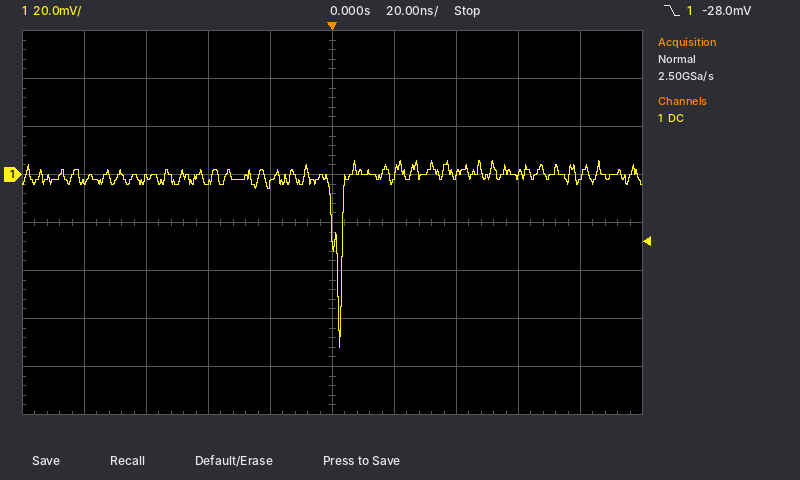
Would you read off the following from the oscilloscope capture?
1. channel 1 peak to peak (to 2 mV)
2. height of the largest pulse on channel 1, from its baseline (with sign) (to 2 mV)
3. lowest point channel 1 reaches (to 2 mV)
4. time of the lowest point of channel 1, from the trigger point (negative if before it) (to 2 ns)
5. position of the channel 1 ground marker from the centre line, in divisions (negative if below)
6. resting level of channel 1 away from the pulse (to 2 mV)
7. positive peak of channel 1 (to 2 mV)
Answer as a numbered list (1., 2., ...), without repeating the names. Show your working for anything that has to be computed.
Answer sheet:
1. 6 mV − (-72 mV) = 78 mV
2. -72 mV − (0 mV) = -72 mV
3. -72 mV
4. +2 ns
5. +1.0 div
6. 0 mV
7. 6 mV
